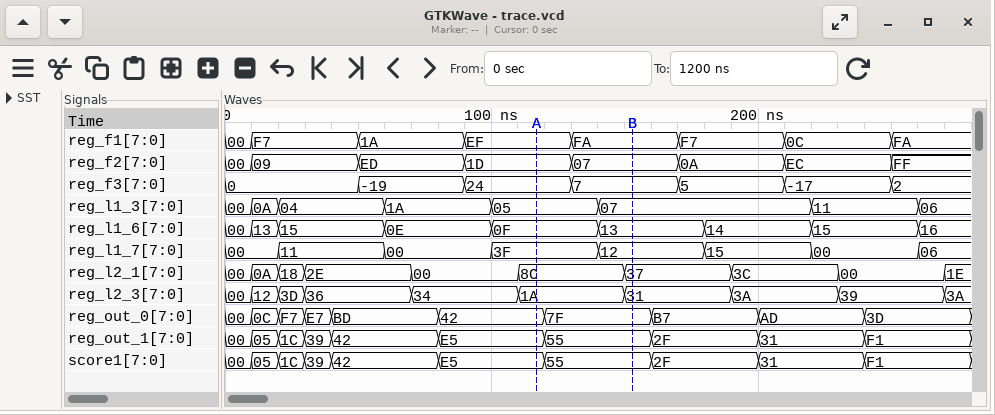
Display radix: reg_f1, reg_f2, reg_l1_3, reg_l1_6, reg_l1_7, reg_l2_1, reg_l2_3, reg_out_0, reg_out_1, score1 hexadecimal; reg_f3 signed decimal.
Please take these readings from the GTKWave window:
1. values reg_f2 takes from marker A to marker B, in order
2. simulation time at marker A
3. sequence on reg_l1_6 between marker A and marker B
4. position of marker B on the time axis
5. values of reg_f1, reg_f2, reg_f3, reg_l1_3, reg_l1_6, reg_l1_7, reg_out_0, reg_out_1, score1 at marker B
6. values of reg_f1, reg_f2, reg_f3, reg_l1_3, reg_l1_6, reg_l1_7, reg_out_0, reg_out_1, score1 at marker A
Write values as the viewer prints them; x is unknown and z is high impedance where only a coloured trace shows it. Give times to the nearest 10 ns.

1D, 07
120 ns
0F, 13
150 ns
reg_f1=FA, reg_f2=07, reg_f3=7, reg_l1_3=07, reg_l1_6=13, reg_l1_7=12, reg_out_0=7F, reg_out_1=55, score1=55
reg_f1=EF, reg_f2=1D, reg_f3=24, reg_l1_3=05, reg_l1_6=0F, reg_l1_7=3F, reg_out_0=42, reg_out_1=E5, score1=E5
